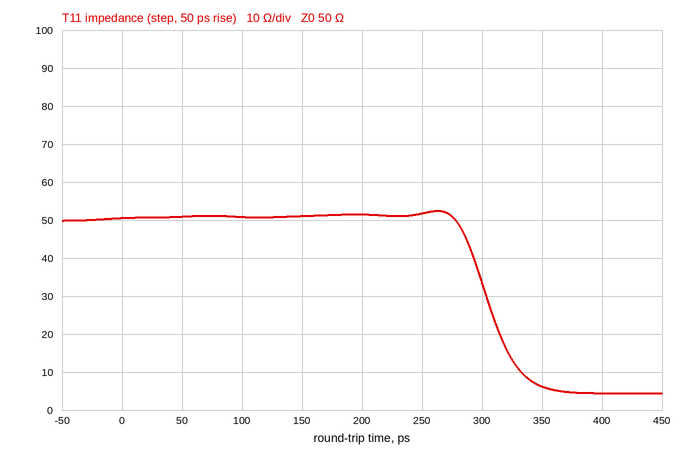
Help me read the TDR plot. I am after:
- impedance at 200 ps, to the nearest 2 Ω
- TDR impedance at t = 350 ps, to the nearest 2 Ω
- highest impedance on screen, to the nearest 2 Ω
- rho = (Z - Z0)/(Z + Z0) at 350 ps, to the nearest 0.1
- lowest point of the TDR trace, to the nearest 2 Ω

52 Ω
6 Ω
52 Ω
-0.8
4 Ω
